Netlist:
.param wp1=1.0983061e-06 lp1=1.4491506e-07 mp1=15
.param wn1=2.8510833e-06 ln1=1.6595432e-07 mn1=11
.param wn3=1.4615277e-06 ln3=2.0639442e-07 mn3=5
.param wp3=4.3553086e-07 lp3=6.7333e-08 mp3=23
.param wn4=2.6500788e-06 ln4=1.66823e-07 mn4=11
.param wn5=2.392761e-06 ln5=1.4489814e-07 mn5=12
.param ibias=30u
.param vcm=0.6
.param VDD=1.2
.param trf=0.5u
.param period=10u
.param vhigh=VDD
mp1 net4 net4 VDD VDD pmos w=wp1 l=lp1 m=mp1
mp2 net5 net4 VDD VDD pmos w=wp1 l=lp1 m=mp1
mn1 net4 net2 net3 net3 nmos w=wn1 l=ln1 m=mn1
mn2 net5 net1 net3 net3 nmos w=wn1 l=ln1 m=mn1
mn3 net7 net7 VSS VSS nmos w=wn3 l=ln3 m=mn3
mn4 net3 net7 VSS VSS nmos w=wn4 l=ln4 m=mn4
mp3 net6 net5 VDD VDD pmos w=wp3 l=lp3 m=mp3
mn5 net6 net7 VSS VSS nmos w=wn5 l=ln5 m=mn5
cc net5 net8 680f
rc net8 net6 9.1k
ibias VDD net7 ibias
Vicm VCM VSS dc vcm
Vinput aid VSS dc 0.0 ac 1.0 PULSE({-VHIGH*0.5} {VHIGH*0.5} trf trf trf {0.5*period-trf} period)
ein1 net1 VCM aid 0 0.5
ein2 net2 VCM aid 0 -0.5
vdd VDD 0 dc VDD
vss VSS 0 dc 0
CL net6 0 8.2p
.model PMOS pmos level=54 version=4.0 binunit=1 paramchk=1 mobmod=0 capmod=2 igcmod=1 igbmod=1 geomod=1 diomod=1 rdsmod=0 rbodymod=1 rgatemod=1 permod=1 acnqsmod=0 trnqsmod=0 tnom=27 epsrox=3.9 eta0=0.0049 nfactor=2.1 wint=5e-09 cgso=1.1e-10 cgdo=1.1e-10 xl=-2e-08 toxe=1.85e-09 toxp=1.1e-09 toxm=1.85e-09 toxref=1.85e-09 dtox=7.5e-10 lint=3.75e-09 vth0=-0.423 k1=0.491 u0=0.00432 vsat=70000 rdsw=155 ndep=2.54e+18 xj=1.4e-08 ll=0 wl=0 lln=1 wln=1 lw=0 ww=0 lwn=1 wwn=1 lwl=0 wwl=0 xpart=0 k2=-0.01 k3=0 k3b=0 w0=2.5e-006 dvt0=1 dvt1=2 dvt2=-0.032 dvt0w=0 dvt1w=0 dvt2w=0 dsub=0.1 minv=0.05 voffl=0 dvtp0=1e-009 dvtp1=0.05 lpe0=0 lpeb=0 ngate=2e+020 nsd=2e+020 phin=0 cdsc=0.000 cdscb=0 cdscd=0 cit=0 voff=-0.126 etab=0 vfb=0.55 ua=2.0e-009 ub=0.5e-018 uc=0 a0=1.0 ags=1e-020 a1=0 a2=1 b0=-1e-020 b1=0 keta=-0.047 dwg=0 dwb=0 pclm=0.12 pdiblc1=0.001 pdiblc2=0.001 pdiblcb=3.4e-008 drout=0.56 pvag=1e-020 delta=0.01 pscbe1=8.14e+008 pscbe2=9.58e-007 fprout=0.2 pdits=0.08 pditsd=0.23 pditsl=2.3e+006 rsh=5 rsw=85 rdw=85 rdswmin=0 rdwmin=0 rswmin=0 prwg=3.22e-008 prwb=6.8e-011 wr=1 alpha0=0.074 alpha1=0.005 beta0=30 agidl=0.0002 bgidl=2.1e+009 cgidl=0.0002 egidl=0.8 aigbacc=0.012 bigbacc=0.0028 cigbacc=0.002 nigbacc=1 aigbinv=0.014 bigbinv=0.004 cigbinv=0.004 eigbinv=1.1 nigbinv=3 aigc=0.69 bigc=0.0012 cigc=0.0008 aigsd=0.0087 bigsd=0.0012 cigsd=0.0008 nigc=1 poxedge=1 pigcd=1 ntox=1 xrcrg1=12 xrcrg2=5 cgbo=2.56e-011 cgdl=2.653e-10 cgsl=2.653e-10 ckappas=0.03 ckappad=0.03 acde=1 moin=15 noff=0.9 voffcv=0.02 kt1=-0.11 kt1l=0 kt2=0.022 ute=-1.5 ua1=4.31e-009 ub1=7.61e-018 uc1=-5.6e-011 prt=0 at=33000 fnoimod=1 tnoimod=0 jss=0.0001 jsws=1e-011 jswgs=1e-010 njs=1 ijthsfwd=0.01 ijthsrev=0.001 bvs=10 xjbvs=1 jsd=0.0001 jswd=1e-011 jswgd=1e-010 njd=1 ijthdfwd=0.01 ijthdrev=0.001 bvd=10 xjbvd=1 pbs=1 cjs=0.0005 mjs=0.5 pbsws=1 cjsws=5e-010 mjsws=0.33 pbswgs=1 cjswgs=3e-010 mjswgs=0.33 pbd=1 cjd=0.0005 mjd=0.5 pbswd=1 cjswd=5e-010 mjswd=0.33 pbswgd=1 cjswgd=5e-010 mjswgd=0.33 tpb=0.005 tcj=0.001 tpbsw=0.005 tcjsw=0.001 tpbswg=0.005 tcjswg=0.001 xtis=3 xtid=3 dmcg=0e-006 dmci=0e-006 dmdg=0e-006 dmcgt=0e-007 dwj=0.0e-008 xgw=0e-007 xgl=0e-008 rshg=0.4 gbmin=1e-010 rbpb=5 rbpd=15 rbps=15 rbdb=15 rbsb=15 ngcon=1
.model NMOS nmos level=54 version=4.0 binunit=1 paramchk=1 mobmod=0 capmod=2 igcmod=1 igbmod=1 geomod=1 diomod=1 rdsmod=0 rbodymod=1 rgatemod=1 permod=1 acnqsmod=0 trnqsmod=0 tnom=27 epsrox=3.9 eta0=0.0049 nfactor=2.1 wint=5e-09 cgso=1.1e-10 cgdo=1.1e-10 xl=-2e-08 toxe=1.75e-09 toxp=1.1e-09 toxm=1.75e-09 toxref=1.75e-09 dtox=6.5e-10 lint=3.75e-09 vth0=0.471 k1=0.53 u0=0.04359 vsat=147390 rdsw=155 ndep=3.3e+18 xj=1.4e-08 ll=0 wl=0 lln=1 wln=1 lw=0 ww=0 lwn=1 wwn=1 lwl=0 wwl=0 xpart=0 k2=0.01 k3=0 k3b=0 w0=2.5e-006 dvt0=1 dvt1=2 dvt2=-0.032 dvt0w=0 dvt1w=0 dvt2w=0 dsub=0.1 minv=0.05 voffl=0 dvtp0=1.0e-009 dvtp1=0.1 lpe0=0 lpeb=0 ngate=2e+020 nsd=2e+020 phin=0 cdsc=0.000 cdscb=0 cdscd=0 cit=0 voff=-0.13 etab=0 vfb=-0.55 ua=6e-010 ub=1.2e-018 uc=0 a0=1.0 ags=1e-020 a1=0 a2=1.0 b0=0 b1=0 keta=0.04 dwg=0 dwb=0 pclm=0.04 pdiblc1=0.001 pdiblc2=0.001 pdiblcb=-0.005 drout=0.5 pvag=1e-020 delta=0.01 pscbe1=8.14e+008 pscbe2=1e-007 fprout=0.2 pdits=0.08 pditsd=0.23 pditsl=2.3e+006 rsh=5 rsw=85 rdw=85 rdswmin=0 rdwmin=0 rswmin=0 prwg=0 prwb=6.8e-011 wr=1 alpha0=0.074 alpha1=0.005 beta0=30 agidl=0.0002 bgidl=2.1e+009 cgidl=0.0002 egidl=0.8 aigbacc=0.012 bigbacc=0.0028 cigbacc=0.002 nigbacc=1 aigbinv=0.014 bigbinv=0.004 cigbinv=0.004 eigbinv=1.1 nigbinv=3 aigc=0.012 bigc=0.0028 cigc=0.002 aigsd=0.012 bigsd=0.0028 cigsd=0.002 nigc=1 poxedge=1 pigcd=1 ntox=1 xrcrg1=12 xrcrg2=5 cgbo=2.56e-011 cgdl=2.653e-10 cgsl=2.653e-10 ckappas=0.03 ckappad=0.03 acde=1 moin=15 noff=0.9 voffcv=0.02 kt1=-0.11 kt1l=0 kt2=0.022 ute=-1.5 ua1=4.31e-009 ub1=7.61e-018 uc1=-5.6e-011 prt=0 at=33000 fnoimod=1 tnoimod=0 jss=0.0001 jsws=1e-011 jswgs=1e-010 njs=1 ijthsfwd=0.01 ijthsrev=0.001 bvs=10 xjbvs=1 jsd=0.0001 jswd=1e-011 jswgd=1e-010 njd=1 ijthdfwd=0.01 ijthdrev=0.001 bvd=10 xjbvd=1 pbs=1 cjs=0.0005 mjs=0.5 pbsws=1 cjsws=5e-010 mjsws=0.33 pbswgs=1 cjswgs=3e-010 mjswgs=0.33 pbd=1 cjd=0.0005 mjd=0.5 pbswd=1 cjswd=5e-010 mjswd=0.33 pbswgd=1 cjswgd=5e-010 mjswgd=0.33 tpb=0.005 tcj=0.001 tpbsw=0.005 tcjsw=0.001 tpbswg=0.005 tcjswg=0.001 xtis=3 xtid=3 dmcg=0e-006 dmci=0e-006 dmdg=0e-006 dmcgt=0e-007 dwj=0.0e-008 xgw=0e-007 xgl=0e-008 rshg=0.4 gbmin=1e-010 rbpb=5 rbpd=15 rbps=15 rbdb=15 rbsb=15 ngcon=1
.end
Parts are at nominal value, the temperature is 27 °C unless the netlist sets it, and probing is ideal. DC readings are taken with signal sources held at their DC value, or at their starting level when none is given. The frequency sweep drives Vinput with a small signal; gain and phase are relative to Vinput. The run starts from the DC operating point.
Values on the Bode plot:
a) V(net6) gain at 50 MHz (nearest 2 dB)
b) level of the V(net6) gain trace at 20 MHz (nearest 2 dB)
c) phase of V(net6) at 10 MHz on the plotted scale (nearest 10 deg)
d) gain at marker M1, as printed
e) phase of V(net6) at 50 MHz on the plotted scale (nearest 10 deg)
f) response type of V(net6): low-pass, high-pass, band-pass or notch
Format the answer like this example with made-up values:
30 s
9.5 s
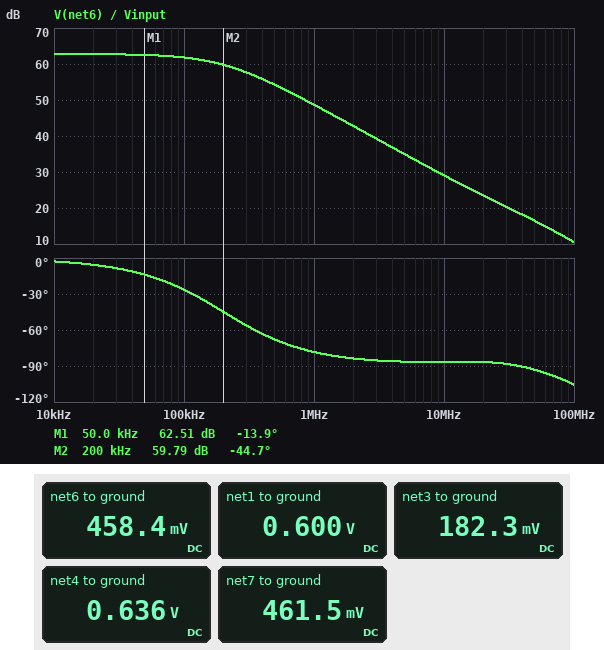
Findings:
16 dB
24 dB
-90 deg
62.51 dB
-90 deg
low-pass
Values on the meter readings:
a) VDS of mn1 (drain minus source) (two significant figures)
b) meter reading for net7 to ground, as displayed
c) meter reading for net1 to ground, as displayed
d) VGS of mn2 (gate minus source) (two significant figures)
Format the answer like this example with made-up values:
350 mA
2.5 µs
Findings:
450 mV
461.5 mV
0.600 V
420 mV
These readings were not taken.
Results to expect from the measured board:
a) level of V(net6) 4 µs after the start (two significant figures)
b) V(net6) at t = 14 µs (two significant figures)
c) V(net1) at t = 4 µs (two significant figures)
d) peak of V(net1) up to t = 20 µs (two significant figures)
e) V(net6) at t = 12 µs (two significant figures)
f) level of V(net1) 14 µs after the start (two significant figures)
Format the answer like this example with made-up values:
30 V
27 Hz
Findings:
1.2 V
1.2 V
900 mV
900 mV
1.2 V
900 mV
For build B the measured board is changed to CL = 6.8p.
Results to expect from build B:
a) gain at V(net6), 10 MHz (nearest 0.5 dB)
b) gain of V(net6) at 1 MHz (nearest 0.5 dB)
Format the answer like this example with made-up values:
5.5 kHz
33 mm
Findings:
29.5 dB
49.0 dB
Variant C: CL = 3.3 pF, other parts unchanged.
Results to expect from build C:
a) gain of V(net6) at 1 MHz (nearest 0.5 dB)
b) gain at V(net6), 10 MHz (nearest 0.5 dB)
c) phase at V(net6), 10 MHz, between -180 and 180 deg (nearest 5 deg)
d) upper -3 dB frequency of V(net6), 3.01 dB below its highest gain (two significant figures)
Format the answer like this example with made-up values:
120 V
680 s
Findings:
49.0 dB
30.0 dB
-75 deg
210 kHz
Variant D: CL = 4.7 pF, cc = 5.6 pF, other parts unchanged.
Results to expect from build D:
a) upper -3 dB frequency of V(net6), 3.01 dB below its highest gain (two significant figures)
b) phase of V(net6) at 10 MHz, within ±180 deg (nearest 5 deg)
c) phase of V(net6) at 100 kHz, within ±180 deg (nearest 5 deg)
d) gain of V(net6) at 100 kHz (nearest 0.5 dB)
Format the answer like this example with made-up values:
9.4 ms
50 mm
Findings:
27 kHz
-30 deg
-75 deg
51.0 dB
